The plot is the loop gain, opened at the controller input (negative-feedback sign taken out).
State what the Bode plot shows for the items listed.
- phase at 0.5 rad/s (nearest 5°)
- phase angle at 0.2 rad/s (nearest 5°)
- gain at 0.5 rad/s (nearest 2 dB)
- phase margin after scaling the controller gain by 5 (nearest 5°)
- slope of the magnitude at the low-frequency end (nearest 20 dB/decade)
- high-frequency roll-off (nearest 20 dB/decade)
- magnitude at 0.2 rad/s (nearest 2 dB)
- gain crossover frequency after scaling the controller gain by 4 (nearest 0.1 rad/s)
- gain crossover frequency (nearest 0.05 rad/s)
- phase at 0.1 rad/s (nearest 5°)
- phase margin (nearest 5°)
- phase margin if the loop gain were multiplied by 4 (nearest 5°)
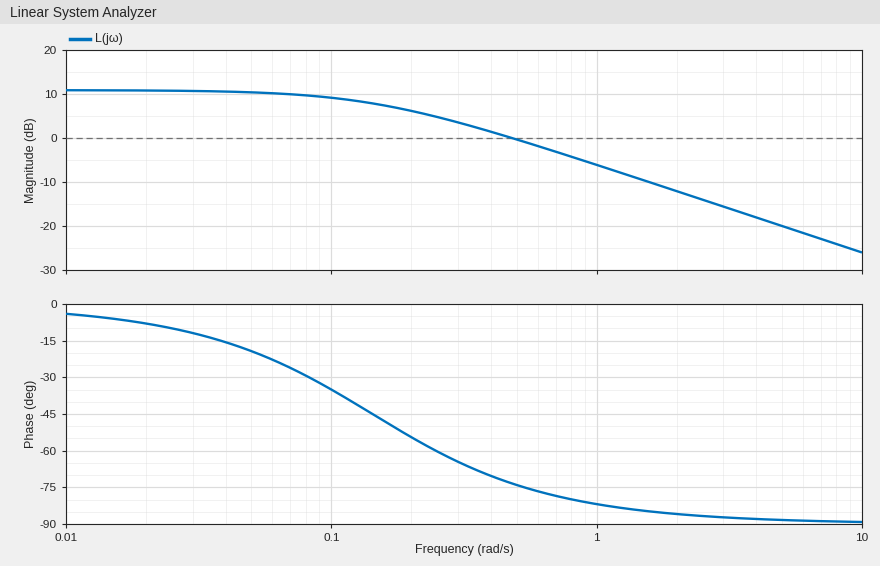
-75°
-55°
0 dB
95°
0 dB/decade
-20 dB/decade
6 dB
2.0 rad/s
0.50 rad/s
-35°
105°
95°
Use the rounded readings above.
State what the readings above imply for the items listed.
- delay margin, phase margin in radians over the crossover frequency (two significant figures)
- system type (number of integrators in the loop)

3.7 s
0
